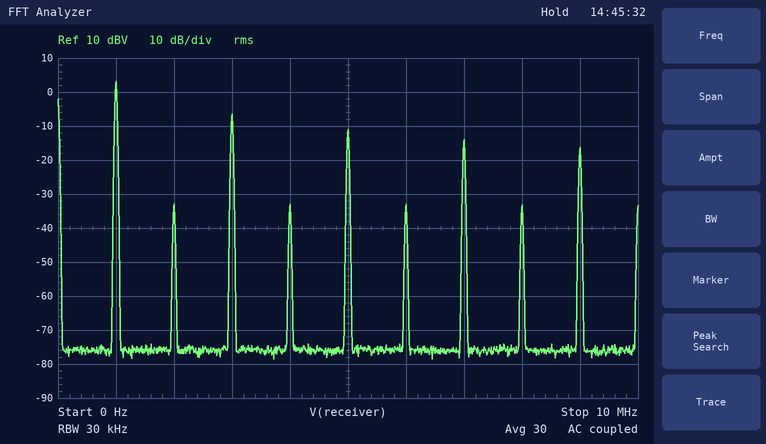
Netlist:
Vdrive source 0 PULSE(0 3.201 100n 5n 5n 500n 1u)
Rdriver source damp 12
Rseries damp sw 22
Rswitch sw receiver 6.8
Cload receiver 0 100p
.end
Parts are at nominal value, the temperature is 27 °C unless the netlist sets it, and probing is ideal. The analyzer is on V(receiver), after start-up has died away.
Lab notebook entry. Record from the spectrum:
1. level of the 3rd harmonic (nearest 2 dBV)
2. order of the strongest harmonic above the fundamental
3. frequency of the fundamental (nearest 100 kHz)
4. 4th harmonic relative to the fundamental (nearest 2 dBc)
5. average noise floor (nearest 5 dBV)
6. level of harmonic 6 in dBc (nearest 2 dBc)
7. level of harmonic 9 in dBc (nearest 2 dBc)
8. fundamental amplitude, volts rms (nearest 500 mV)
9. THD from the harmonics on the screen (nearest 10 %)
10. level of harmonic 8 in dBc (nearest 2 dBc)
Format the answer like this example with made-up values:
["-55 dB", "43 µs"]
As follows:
["-6 dBV", "3", "1.0 MHz", "-36 dBc", "-75 dBV", "-36 dBc", "-20 dBc", "1.5 V", "40 %", "-36 dBc"]
